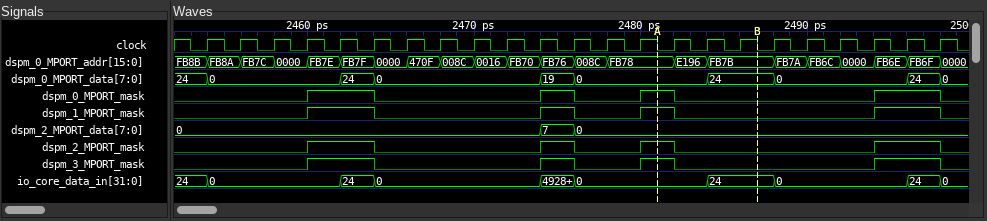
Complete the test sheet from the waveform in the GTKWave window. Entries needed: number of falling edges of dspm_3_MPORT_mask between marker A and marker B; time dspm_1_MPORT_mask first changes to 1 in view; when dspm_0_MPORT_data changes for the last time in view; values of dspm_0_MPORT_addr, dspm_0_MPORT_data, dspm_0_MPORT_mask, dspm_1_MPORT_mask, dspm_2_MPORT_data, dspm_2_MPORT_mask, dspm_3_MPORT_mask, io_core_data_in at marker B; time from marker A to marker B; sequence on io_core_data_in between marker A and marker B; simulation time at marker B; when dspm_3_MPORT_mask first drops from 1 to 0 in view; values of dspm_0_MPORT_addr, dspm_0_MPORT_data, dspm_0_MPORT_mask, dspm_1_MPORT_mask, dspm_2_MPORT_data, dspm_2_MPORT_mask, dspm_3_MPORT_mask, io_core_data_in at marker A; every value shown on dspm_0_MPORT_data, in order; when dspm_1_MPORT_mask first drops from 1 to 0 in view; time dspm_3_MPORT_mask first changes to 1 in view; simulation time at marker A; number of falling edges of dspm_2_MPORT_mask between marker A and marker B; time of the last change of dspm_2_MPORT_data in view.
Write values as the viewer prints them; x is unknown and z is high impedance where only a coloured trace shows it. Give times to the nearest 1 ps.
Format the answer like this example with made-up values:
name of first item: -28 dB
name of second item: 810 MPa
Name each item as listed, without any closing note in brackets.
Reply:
number of falling edges of dspm_3_MPORT_mask between marker A and marker B: 1
time dspm_1_MPORT_mask first changes to 1 in view: 2460 ps
when dspm_0_MPORT_data changes for the last time in view: 2498 ps
values of dspm_0_MPORT_addr, dspm_0_MPORT_data, dspm_0_MPORT_mask, dspm_1_MPORT_mask, dspm_2_MPORT_data, dspm_2_MPORT_mask, dspm_3_MPORT_mask, io_core_data_in at marker B: dspm_0_MPORT_addr=FB7B, dspm_0_MPORT_data=24, dspm_0_MPORT_mask=0, dspm_1_MPORT_mask=0, dspm_2_MPORT_data=0, dspm_2_MPORT_mask=0, dspm_3_MPORT_mask=0, io_core_data_in=24
time from marker A to marker B: 6 ps
sequence on io_core_data_in between marker A and marker B: 0, 24
simulation time at marker B: 2487 ps
when dspm_3_MPORT_mask first drops from 1 to 0 in view: 2464 ps
values of dspm_0_MPORT_addr, dspm_0_MPORT_data, dspm_0_MPORT_mask, dspm_1_MPORT_mask, dspm_2_MPORT_data, dspm_2_MPORT_mask, dspm_3_MPORT_mask, io_core_data_in at marker A: dspm_0_MPORT_addr=FB78, dspm_0_MPORT_data=0, dspm_0_MPORT_mask=1, dspm_1_MPORT_mask=1, dspm_2_MPORT_data=0, dspm_2_MPORT_mask=1, dspm_3_MPORT_mask=1, io_core_data_in=0
every value shown on dspm_0_MPORT_data, in order: 24, 0, 24, 0, 19, 0, 24, 0, 24, 0
when dspm_1_MPORT_mask first drops from 1 to 0 in view: 2464 ps
time dspm_3_MPORT_mask first changes to 1 in view: 2460 ps
simulation time at marker A: 2481 ps
number of falling edges of dspm_2_MPORT_mask between marker A and marker B: 1
time of the last change of dspm_2_MPORT_data in view: 2476 ps
